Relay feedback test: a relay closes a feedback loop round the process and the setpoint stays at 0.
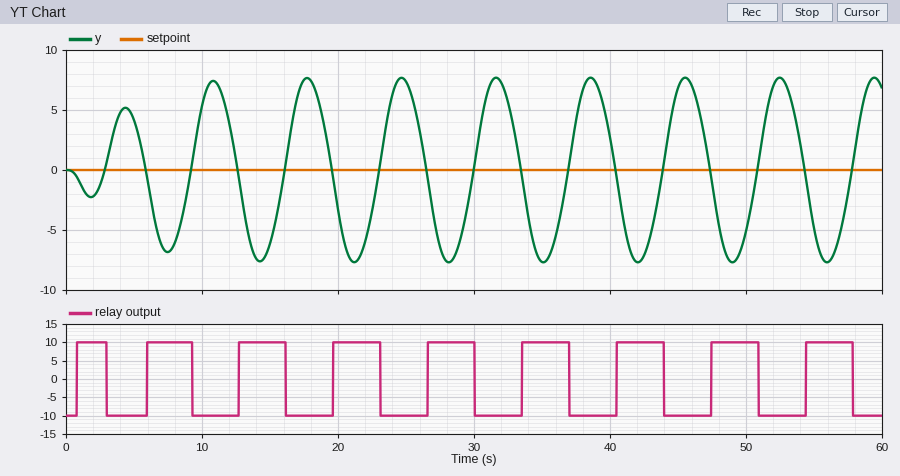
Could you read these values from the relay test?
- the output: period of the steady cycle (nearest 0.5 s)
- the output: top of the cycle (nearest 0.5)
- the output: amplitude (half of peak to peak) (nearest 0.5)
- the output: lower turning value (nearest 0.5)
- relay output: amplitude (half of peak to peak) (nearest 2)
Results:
7.0 s
7.5
7.5
-7.5
10
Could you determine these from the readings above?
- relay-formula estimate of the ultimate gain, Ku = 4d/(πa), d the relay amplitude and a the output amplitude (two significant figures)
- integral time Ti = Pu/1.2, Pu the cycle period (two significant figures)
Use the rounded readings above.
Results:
1.7
5.8 s
